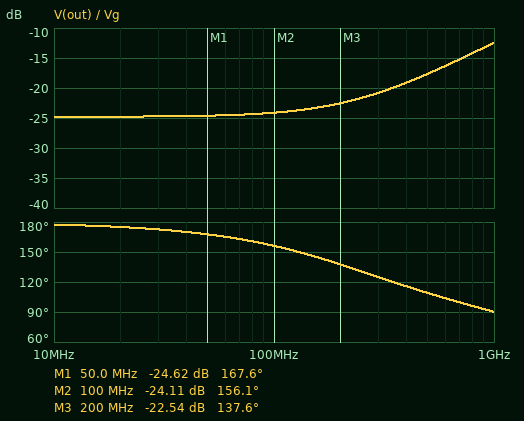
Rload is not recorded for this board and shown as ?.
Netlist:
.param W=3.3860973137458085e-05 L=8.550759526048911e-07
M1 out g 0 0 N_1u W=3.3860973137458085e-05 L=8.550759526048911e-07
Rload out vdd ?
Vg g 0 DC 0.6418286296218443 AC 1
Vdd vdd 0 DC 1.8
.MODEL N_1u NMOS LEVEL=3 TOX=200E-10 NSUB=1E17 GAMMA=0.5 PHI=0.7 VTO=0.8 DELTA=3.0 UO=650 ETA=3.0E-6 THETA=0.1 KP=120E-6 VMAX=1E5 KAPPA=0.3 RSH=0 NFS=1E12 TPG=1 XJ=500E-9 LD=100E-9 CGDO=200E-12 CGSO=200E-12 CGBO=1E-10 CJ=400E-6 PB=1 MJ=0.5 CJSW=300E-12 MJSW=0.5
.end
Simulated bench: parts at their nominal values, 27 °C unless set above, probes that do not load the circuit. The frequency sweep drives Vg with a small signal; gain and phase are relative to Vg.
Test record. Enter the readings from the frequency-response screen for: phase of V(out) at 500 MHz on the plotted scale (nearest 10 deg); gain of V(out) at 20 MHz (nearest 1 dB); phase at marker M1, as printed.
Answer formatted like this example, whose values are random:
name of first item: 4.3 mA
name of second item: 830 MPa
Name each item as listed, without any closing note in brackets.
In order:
phase of V(out) at 500 MHz on the plotted scale: 110 deg
gain of V(out) at 20 MHz: -25 dB
phase at marker M1, as printed: 167.6 deg
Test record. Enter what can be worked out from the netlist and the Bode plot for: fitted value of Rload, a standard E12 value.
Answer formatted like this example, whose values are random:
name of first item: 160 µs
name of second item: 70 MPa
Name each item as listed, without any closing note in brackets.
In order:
fitted value of Rload, a standard E12 value: 5.6 kΩ
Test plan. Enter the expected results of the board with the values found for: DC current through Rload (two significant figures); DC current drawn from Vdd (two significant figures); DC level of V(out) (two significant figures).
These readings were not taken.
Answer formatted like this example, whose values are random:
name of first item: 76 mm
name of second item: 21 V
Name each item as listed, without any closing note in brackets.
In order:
DC current through Rload: 580 nA
DC current drawn from Vdd: 580 nA
DC level of V(out): 1.8 V
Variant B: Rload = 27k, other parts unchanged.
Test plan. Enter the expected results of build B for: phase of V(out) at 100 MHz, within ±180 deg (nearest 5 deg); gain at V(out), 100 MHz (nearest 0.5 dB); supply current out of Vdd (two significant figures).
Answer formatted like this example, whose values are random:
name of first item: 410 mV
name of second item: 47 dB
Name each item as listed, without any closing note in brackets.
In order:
phase of V(out) at 100 MHz, within ±180 deg: 150 deg
gain at V(out), 100 MHz: -10.5 dB
supply current out of Vdd: 580 nA
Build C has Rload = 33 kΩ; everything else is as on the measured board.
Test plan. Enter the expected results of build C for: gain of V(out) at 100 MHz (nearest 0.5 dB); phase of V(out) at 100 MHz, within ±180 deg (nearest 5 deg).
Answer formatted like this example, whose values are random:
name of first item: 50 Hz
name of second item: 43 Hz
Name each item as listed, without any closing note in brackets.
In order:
gain of V(out) at 100 MHz: -9.0 dB
phase of V(out) at 100 MHz, within ±180 deg: 150 deg
